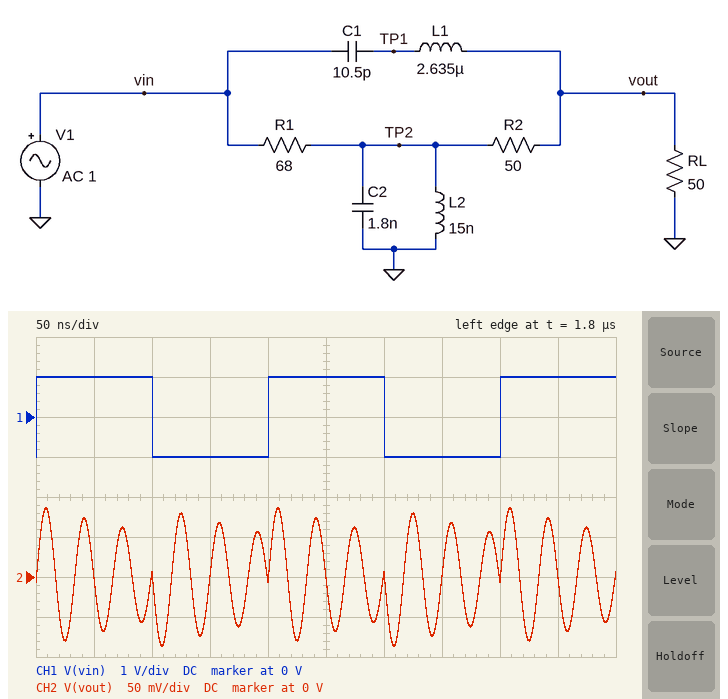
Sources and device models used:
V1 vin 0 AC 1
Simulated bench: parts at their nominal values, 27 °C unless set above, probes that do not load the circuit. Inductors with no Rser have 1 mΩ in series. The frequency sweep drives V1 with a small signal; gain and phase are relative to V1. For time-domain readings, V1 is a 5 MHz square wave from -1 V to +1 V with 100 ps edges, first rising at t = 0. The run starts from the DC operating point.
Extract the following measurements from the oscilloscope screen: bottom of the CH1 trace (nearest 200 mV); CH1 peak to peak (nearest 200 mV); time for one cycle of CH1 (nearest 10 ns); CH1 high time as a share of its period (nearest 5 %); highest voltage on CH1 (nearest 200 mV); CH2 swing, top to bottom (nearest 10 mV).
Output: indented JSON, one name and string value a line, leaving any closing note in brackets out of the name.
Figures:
{
  "bottom of the CH1 trace": "-1.0 V",
  "CH1 peak to peak": "2.0 V",
  "time for one cycle of CH1": "200 ns",
  "CH1 high time as a share of its period": "50 %",
  "highest voltage on CH1": "1.0 V",
  "CH2 swing, top to bottom": "170 mV"
}
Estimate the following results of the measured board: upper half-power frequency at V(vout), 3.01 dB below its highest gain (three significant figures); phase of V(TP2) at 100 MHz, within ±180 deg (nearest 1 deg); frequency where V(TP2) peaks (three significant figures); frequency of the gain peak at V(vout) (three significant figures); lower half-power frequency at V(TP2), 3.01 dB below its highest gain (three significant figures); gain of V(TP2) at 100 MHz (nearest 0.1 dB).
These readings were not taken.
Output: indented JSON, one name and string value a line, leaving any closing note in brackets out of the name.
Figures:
{
  "upper half-power frequency at V(vout), 3.01 dB below its highest gain": "31.7 MHz",
  "phase of V(TP2) at 100 MHz, within ±180 deg": "-90 deg",
  "frequency where V(TP2) peaks": "30.4 MHz",
  "frequency of the gain peak at V(vout)": "30.0 MHz",
  "lower half-power frequency at V(TP2), 3.01 dB below its highest gain": "29.4 MHz",
  "gain of V(TP2) at 100 MHz": "-36.9 dB"
}
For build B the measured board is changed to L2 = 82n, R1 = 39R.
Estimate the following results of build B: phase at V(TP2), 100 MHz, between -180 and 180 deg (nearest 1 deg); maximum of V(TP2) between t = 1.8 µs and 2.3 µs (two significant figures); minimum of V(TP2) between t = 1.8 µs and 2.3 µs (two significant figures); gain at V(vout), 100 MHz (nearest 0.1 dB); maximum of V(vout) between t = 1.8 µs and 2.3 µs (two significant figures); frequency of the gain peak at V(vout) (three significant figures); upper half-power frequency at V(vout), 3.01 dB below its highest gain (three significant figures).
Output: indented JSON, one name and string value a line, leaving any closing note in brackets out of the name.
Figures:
{
  "phase at V(TP2), 100 MHz, between -180 and 180 deg": "-89 deg",
  "maximum of V(TP2) between t = 1.8 µs and 2.3 µs": "290 mV",
  "minimum of V(TP2) between t = 1.8 µs and 2.3 µs": "-290 mV",
  "gain at V(vout), 100 MHz": "-31.0 dB",
  "maximum of V(vout) between t = 1.8 µs and 2.3 µs": "140 mV",
  "frequency of the gain peak at V(vout)": "30.3 MHz",
  "upper half-power frequency at V(vout), 3.01 dB below its highest gain": "31.1 MHz"
}
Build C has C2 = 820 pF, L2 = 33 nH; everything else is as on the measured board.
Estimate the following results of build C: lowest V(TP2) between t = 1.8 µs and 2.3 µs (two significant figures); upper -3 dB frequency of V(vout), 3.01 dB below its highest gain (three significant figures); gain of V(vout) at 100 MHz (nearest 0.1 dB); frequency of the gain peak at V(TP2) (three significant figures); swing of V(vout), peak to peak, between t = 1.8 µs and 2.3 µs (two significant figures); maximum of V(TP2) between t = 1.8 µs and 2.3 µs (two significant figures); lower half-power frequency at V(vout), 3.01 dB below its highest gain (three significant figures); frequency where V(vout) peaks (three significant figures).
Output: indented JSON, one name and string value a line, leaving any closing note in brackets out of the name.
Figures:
{
  "lowest V(TP2) between t = 1.8 µs and 2.3 µs": "-120 mV",
  "upper -3 dB frequency of V(vout), 3.01 dB below its highest gain": "31.8 MHz",
  "gain of V(vout) at 100 MHz": "-29.8 dB",
  "frequency of the gain peak at V(TP2)": "30.2 MHz",
  "swing of V(vout), peak to peak, between t = 1.8 µs and 2.3 µs": "260 mV",
  "maximum of V(TP2) between t = 1.8 µs and 2.3 µs": "120 mV",
  "lower half-power frequency at V(vout), 3.01 dB below its highest gain": "28.8 MHz",
  "frequency where V(vout) peaks": "30.1 MHz"
}
